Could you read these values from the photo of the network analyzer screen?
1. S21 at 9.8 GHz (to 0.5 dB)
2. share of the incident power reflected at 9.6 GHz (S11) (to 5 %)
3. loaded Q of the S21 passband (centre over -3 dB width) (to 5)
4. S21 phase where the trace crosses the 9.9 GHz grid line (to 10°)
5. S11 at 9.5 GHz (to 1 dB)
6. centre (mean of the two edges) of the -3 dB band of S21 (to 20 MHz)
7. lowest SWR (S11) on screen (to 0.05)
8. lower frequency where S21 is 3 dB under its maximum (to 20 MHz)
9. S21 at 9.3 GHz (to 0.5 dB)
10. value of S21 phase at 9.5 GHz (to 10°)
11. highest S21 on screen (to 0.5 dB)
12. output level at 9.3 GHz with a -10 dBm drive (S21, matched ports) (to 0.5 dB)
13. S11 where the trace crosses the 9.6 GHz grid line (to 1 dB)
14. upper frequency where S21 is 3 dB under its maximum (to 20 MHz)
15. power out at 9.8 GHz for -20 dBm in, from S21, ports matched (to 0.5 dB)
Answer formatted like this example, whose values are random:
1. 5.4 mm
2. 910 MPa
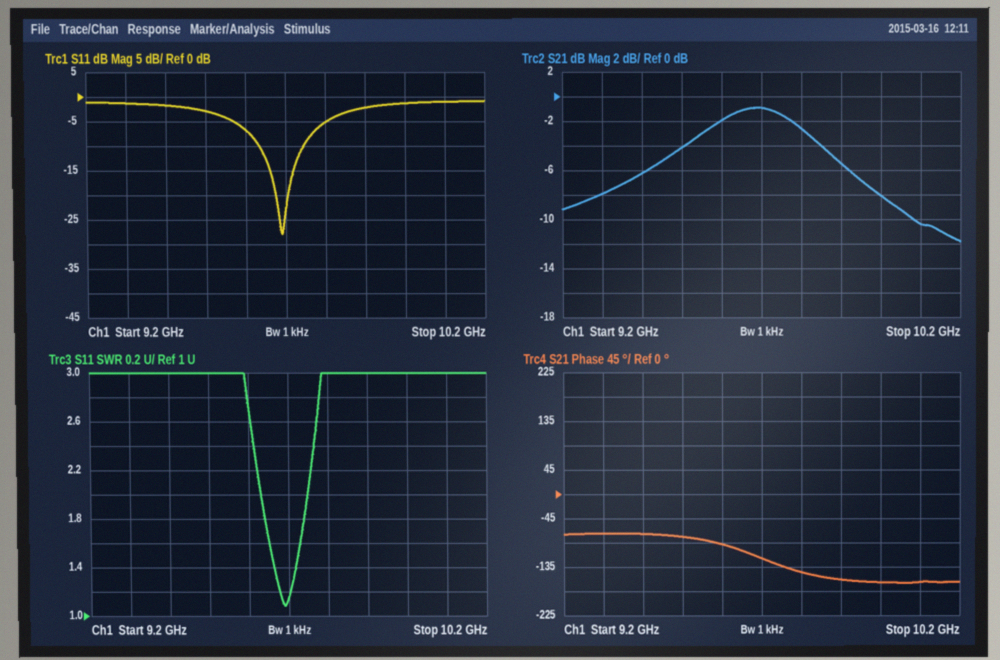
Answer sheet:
1. -2.5 dB
2. 20 %
3. 30
4. -160°
5. -3 dB
6. 9.68 GHz
7. 1.10
8. 9.52 GHz
9. -8.0 dB
10. -80°
11. -1.0 dB
12. -18.0 dBm
13. -7 dB
14. 9.84 GHz
15. -22.5 dBm
